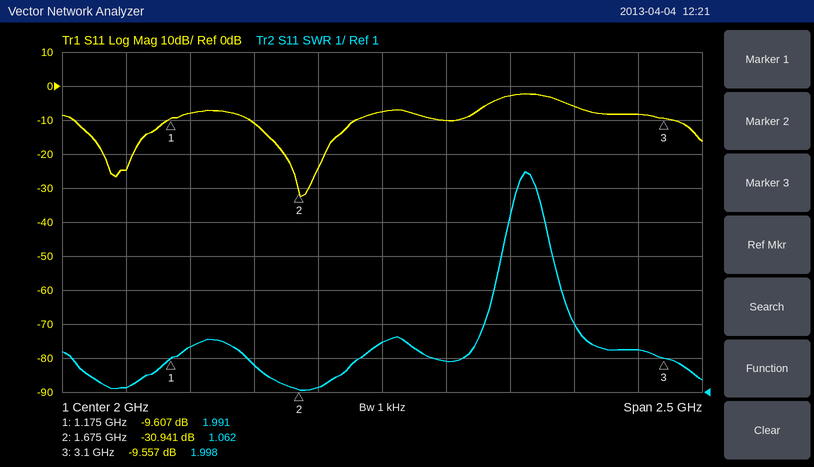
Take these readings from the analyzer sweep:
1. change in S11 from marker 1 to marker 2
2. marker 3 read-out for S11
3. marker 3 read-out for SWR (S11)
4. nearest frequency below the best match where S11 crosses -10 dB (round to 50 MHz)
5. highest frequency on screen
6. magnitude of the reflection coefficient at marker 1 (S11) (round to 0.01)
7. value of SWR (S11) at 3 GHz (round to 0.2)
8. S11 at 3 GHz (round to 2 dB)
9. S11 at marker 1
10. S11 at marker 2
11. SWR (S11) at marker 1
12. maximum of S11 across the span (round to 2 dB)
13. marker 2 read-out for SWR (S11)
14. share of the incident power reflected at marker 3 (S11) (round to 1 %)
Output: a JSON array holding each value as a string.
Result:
["-21.334 dB", "-9.557 dB", "1.998", "1.50 GHz", "3.25 GHz", "0.33", "2.2", "-8 dB", "-9.607 dB", "-30.941 dB", "1.991", "-2 dB", "1.062", "11 %"]
